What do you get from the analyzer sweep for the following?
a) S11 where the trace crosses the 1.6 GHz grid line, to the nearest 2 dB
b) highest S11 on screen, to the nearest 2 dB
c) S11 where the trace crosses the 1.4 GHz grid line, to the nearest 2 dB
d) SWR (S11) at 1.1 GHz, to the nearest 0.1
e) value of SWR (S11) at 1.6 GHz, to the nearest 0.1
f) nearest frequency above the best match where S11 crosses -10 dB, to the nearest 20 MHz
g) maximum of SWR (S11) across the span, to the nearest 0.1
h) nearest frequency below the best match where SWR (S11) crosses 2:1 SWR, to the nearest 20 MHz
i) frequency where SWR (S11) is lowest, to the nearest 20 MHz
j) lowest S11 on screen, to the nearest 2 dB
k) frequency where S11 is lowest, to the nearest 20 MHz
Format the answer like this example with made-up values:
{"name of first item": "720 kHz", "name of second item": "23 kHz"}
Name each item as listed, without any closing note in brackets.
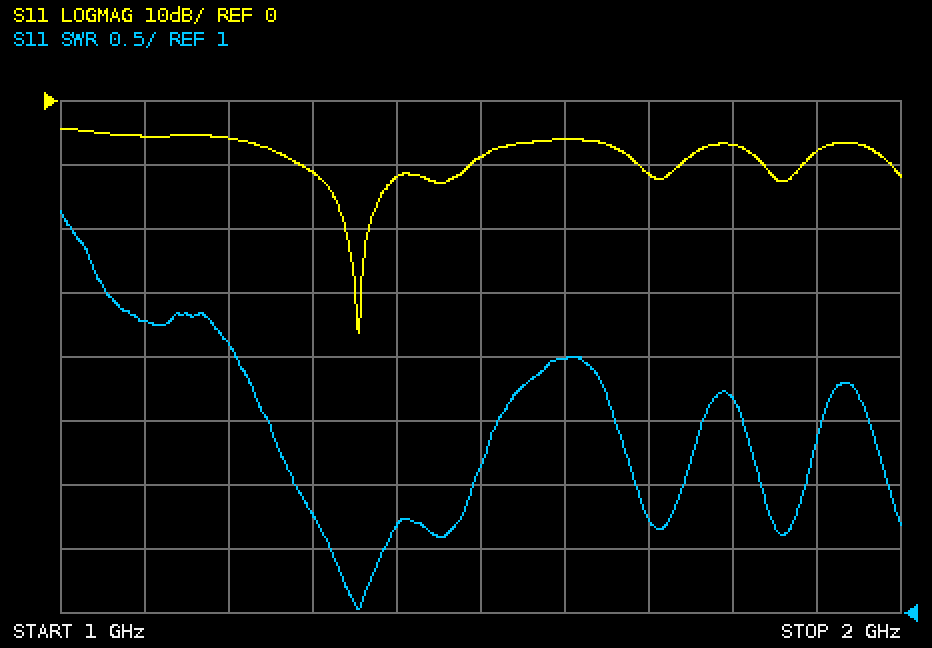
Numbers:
{"S11 where the trace crosses the 1.6 GHz grid line, to the nearest 2 dB": "-6 dB", "highest S11 on screen, to the nearest 2 dB": "-4 dB", "S11 where the trace crosses the 1.4 GHz grid line, to the nearest 2 dB": "-12 dB", "SWR (S11) at 1.1 GHz, to the nearest 0.1": "3.3", "value of SWR (S11) at 1.6 GHz, to the nearest 0.1": "3.0", "nearest frequency above the best match where S11 crosses -10 dB, to the nearest 20 MHz": "1.48 GHz", "maximum of SWR (S11) across the span, to the nearest 0.1": "4.1", "nearest frequency below the best match where SWR (S11) crosses 2:1 SWR, to the nearest 20 MHz": "1.28 GHz", "frequency where SWR (S11) is lowest, to the nearest 20 MHz": "1.36 GHz", "lowest S11 on screen, to the nearest 2 dB": "-36 dB", "frequency where S11 is lowest, to the nearest 20 MHz": "1.36 GHz"}
